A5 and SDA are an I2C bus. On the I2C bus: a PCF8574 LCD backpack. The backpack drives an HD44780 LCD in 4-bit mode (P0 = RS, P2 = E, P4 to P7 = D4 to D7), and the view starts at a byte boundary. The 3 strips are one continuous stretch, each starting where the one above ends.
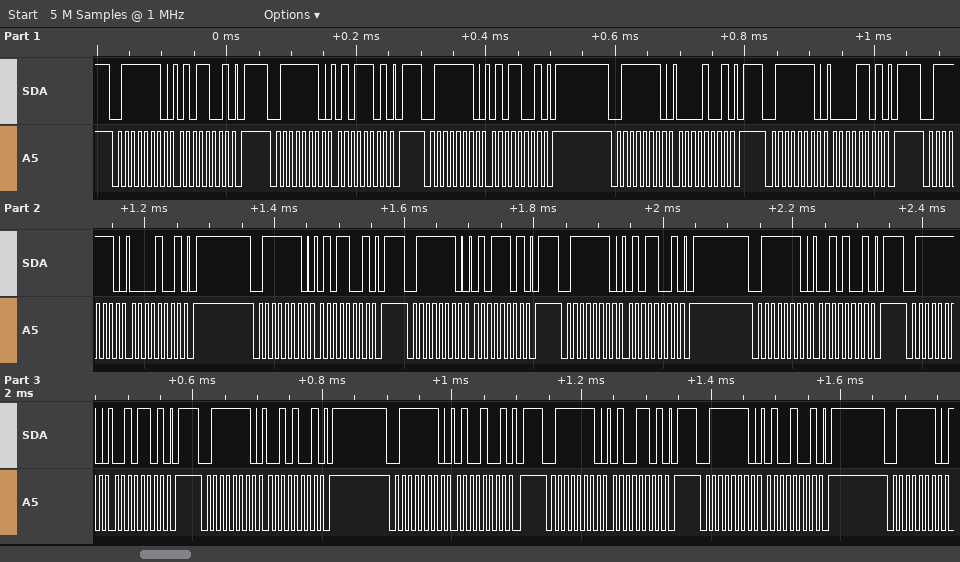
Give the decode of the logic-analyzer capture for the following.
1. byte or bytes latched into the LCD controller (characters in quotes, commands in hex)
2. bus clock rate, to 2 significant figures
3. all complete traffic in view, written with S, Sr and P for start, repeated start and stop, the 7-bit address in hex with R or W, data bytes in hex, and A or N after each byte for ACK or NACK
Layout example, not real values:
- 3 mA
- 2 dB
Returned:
- 'P' 'R'
- 100 kHz
- S 3FW A 59 A P S 3FW A 5D A P S 3FW A 59 A P S 3FW A 09 A P S 3FW A 0D A P S 3FW A 09 A P S 3FW A 59 A P S 3FW A 5D A P S 3FW A 59 A P S 3FW A 29 A P S 3FW A 2D A P S 3FW A 29 A P S 3FW A 49 A P S 3FW A 4D A P S 3FW A 49 A P S 3FW A
